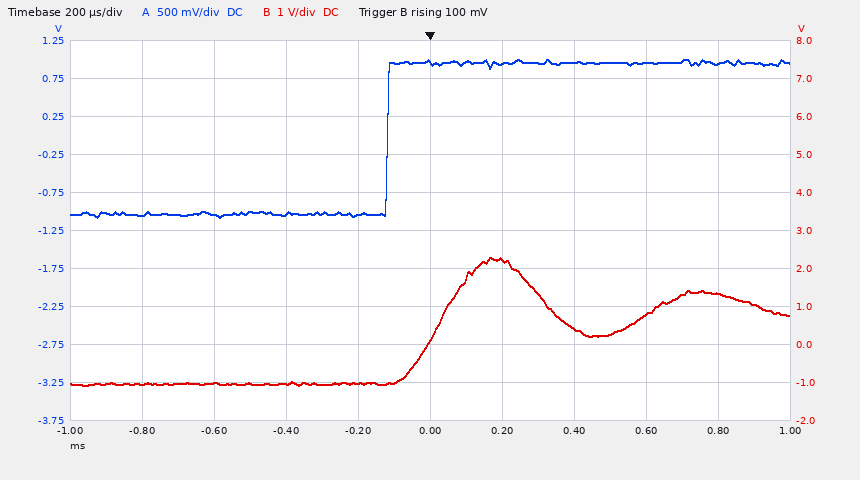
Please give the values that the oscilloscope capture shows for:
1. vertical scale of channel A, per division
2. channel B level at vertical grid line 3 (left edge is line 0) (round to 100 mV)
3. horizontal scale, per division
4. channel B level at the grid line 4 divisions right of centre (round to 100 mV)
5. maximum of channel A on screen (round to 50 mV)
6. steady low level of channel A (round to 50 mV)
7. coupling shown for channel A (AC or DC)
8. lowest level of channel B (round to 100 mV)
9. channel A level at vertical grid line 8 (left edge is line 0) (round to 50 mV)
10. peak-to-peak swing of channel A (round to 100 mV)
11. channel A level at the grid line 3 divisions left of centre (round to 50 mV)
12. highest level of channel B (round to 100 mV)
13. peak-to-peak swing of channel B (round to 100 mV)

500 mV
-1.0 V
200 µs
1.3 V
1.00 V
-1.05 V
DC
-1.1 V
950 mV
2.10 V
-1.05 V
2.3 V
3.4 V
